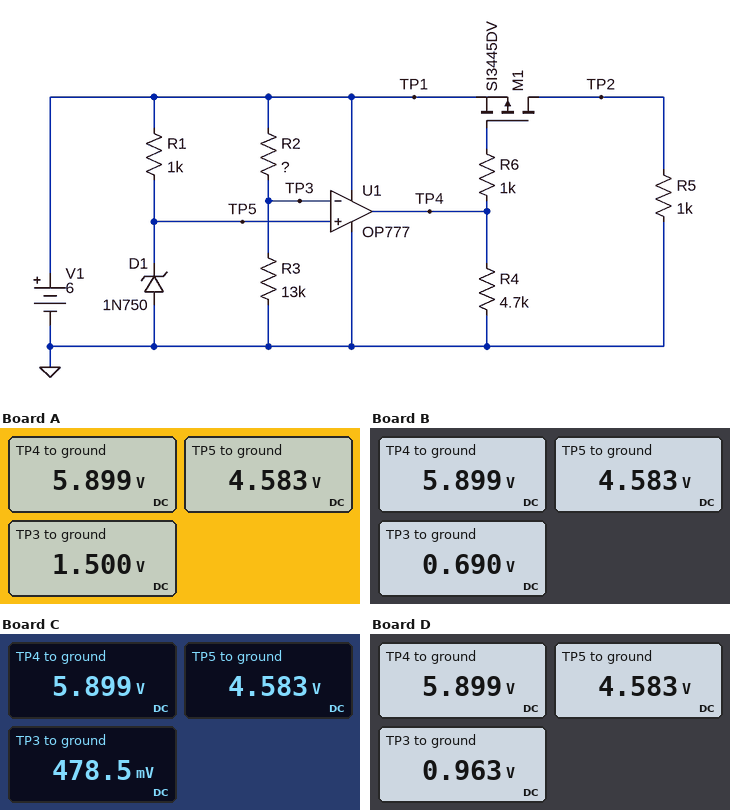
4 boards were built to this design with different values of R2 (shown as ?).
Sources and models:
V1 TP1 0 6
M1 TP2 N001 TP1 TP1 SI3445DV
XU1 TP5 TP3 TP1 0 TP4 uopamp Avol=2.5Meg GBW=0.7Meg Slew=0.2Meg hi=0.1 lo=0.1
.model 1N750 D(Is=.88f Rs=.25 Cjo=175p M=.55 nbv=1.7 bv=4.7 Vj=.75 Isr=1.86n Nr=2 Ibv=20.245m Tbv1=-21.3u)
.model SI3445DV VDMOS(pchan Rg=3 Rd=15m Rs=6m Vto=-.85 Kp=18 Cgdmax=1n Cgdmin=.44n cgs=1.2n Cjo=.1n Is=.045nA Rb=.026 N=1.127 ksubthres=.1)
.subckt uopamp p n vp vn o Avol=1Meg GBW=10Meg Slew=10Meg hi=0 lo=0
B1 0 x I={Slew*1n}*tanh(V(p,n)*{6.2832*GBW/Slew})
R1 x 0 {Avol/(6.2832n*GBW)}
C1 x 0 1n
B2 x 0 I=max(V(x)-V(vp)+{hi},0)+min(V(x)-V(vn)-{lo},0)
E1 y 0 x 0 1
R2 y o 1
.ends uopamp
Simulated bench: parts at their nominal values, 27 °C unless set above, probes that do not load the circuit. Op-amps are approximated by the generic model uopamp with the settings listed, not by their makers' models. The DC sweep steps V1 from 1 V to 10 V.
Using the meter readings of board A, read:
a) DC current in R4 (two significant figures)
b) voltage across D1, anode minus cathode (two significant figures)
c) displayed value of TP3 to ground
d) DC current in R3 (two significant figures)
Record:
1.3 mA
-4.6 V
1.500 V
120 µA
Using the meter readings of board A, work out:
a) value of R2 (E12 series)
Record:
39 kΩ
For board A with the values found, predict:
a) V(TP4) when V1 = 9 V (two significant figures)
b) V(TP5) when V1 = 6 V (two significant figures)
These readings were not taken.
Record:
8.9 V
4.6 V
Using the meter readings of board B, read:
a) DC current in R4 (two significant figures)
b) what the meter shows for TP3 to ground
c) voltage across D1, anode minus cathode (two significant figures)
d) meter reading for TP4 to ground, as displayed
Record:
1.3 mA
0.690 V
-4.6 V
5.899 V
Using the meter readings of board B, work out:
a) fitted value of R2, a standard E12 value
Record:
100 kΩ
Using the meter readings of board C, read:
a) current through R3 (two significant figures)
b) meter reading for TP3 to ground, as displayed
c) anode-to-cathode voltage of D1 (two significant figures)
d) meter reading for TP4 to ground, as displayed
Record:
37 µA
478.5 mV
-4.6 V
5.899 V
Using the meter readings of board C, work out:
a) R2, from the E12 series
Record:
150 kΩ
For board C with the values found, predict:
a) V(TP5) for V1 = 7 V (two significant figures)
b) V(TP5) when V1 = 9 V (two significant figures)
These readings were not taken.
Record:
4.6 V
4.6 V
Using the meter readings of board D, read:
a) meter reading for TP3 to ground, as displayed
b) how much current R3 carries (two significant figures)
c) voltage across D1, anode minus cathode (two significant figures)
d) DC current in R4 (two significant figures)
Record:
0.963 V
74 µA
-4.6 V
1.3 mA
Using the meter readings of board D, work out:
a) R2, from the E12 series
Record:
68 kΩ
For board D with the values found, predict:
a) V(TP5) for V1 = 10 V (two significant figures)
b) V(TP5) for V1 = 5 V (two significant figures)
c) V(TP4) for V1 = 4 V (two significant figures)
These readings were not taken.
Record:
4.6 V
4.5 V
3.9 V
